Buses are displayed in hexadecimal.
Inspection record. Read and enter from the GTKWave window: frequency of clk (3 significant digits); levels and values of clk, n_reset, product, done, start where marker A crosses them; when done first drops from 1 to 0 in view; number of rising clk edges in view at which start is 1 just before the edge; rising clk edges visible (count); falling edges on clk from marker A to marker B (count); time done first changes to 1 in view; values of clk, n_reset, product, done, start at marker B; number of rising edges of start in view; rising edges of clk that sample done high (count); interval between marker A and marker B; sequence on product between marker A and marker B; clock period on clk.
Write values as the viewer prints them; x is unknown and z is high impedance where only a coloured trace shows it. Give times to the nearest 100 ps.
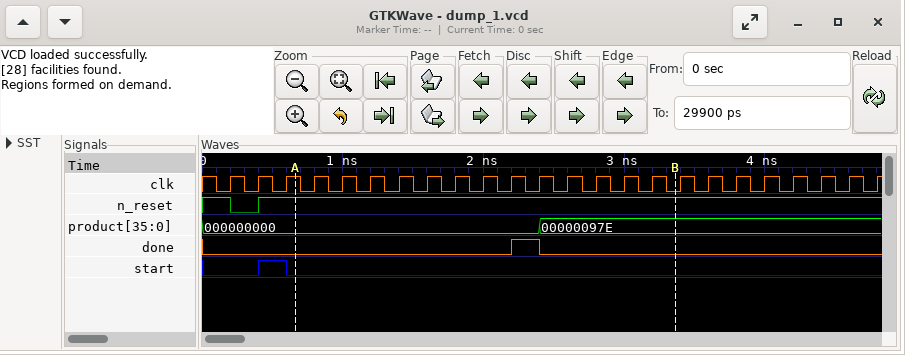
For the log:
5.00 GHz
clk=1, n_reset=1, product=000000000, done=0, start=0
2400 ps
1
24
14
2200 ps
clk=0, n_reset=1, product=00000097E, done=0, start=0
1
1
2700 ps
000000000, 00000097E
200 ps
